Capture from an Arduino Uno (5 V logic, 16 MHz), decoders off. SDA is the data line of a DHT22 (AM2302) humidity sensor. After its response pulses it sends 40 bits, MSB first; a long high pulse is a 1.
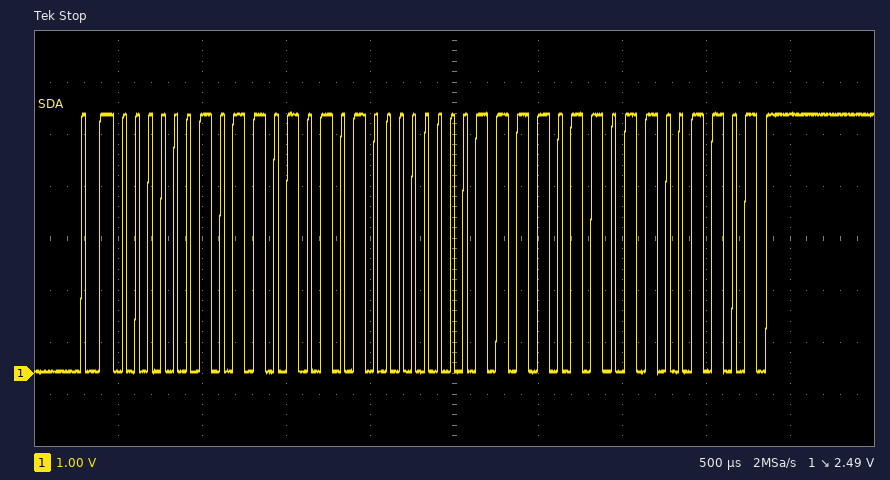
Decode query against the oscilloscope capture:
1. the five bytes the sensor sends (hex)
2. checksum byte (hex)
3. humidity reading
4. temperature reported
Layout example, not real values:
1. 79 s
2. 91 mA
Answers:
1. 02 D5 00 F6 CD
2. 0xCD
3. 72.5 %
4. 24.6 °C
